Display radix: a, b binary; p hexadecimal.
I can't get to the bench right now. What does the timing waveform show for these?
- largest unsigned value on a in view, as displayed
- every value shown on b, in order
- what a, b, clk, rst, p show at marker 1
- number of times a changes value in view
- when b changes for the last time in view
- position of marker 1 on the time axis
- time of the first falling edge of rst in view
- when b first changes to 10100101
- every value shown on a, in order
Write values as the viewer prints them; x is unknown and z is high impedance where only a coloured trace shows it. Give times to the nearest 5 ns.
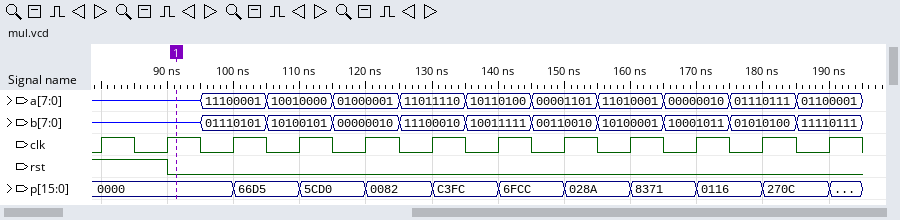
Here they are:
11100001
z, 01110101, 10100101, 00000010, 11100010, 10011111, 00110010, 10100001, 10001011, 01010100, 11110111
a=z, b=z, clk=1, rst=0, p=0000
10
185 ns
90 ns
90 ns
105 ns
z, 11100001, 10010000, 01000001, 11011110, 10110100, 00001101, 11010001, 00000010, 01110111, 01100001
